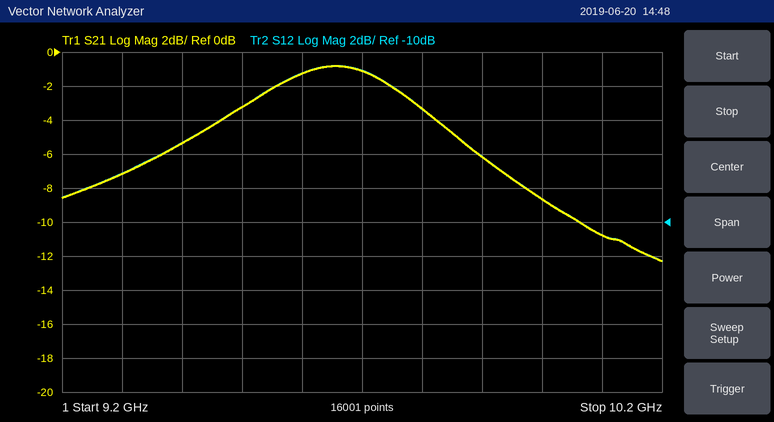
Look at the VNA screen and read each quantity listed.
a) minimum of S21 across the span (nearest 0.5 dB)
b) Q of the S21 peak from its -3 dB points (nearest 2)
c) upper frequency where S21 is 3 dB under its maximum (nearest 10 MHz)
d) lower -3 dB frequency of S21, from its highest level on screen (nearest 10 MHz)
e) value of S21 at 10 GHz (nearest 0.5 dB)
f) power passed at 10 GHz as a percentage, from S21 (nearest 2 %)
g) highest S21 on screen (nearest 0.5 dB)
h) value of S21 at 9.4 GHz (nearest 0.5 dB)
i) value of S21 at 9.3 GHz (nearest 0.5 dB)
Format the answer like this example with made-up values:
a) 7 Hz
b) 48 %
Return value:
a) -12.5 dB
b) 28
c) 9.82 GHz
d) 9.47 GHz
e) -8.5 dB
f) 14 %
g) -1.0 dB
h) -5.5 dB
i) -7.0 dB
